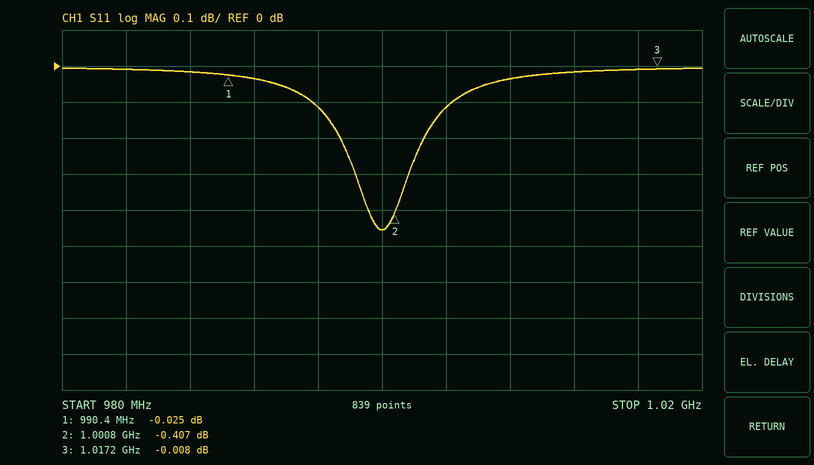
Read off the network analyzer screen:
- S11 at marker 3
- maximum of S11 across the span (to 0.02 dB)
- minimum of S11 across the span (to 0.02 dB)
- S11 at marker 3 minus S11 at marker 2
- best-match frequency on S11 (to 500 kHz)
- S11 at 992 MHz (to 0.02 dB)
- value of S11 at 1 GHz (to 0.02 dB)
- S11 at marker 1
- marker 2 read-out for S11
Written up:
-0.008 dB
0.00 dB
-0.46 dB
0.399 dB
1.0000 GHz
-0.04 dB
-0.46 dB
-0.025 dB
-0.407 dB
